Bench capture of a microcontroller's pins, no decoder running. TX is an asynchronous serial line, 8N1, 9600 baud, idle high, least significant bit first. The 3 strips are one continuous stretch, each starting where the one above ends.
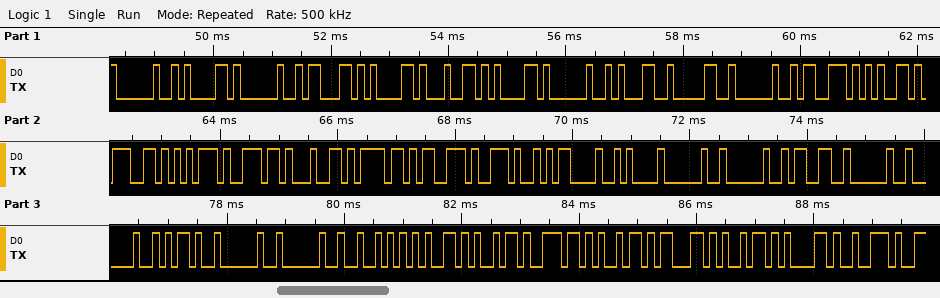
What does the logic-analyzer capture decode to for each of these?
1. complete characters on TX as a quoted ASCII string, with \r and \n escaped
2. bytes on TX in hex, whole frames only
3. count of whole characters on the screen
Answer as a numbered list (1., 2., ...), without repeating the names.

1. " a cada 10 segundos.\r\n  3  -  Reiniciar"
2. 20 61 20 63 61 64 61 20 31 30 20 73 65 67 75 6E 64 6F 73 2E 0D 0A 20 20 33 20 20 2D 20 20 52 65 69 6E 69 63 69 61 72
3. 39
